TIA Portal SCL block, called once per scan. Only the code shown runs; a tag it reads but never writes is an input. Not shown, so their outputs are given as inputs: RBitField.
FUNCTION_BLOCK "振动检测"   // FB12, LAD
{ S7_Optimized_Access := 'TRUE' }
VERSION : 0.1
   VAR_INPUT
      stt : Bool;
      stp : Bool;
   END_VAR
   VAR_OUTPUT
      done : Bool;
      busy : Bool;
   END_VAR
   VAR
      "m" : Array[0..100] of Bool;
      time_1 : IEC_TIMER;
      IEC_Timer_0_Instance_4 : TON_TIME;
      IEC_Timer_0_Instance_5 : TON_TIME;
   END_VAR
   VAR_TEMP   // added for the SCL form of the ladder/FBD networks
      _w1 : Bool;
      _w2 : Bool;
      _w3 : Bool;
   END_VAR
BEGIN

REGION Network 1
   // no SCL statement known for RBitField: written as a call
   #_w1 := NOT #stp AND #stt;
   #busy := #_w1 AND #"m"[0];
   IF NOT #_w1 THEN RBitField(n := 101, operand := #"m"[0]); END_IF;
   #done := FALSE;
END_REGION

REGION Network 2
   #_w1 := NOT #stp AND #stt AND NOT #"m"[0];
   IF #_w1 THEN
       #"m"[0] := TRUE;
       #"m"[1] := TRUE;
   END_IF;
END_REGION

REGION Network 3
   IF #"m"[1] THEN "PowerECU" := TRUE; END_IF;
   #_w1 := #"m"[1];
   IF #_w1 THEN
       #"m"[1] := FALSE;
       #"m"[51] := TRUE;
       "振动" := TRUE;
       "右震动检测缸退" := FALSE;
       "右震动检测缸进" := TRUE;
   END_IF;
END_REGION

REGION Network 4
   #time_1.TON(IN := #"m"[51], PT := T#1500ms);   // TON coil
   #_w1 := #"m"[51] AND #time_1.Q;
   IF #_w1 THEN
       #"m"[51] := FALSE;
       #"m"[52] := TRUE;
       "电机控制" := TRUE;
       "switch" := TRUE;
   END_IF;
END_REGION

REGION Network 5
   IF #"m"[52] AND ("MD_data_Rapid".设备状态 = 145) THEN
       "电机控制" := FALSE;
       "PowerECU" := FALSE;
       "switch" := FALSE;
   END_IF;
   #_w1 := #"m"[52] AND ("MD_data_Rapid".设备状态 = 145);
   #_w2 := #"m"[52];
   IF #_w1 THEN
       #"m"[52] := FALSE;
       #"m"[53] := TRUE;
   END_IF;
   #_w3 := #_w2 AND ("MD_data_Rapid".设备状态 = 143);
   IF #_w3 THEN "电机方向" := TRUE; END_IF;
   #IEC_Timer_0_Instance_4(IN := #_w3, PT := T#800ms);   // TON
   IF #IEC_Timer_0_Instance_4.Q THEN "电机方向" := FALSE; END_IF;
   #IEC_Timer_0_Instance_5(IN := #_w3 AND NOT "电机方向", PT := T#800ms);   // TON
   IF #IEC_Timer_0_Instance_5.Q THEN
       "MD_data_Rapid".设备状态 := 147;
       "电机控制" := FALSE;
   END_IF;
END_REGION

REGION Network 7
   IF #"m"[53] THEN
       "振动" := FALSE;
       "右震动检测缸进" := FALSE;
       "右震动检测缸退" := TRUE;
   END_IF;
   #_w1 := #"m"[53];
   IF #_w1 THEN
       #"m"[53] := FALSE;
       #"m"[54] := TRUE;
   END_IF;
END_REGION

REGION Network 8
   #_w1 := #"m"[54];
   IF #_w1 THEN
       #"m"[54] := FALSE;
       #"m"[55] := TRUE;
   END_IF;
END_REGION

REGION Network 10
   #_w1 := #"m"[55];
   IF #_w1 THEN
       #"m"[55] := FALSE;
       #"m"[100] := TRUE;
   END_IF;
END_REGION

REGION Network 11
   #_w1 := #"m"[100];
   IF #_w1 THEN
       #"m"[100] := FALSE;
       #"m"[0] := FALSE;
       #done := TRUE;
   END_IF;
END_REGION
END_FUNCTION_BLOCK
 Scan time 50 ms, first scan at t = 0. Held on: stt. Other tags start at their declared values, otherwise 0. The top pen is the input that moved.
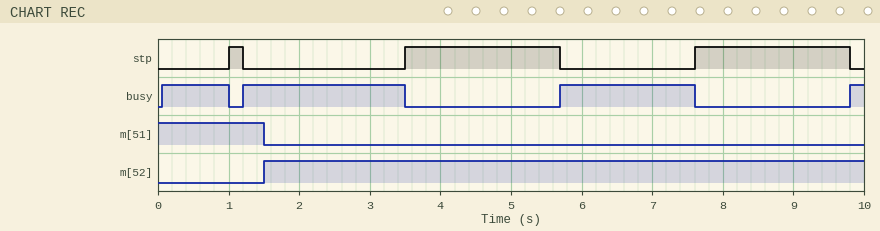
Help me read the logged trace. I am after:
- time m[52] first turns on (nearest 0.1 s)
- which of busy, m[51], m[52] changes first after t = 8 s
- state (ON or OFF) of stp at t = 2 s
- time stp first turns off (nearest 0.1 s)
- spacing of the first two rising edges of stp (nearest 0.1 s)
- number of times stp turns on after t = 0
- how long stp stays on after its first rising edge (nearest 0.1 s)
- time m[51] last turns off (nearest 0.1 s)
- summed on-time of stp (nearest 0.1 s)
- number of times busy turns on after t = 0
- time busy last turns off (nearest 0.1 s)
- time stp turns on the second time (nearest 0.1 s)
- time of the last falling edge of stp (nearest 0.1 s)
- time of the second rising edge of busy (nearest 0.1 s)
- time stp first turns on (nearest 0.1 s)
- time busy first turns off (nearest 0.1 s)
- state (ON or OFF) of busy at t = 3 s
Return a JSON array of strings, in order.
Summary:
["1.5 s", "busy", "OFF", "1.2 s", "2.5 s", "3", "0.2 s", "1.5 s", "4.6 s", "4", "7.6 s", "3.5 s", "9.8 s", "1.2 s", "1.0 s", "1.0 s", "ON"]
